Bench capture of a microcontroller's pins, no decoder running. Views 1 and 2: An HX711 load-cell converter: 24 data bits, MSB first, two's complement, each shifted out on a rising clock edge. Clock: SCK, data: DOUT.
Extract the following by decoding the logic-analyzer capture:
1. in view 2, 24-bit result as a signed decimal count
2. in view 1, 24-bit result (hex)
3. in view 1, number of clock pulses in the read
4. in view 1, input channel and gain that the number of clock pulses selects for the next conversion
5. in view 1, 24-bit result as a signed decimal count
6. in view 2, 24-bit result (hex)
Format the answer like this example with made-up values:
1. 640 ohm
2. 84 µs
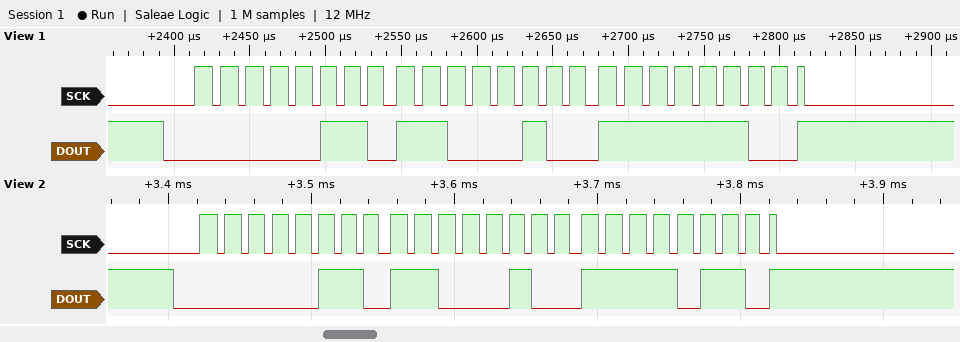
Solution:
1. 443638
2. 0x06C4FC
3. 25
4. channel A, gain 128
5. 443644
6. 0x06C4F6
